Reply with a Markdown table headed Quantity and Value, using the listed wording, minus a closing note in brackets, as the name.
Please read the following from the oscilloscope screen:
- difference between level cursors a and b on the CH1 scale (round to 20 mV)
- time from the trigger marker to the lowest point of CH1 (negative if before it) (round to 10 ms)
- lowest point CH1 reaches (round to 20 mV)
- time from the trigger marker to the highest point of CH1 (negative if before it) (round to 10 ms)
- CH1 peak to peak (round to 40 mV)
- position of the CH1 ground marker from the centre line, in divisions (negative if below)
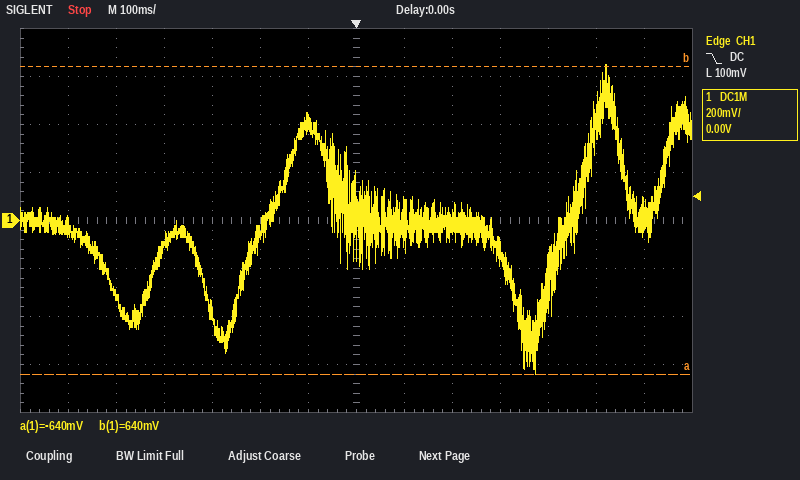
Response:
| Quantity | Value |
|---|---|
| difference between level cursors a and b on the CH1 scale | 1.28 V |
| time from the trigger marker to the lowest point of CH1 (negative if before it) | +370 ms |
| lowest point CH1 reaches | -640 mV |
| time from the trigger marker to the highest point of CH1 (negative if before it) | +520 ms |
| CH1 peak to peak | 1.28 V |
| position of the CH1 ground marker from the centre line, in divisions | 0.0 div |
